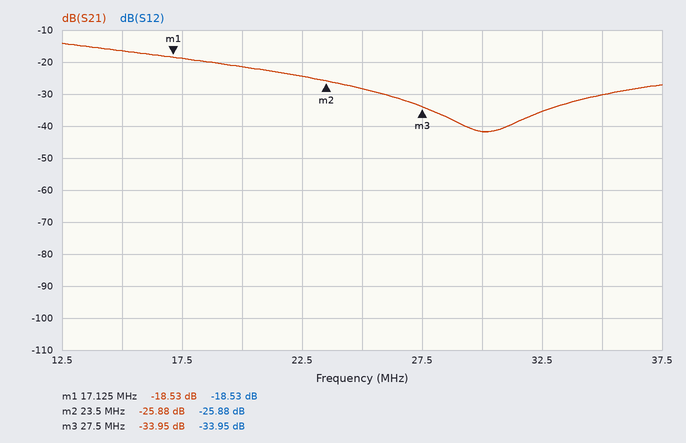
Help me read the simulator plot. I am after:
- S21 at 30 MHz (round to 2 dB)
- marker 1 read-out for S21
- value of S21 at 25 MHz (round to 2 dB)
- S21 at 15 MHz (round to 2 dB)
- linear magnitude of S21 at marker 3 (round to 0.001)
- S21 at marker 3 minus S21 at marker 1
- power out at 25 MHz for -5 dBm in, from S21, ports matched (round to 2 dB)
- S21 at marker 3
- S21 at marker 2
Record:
-42 dB
-18.53 dB
-28 dB
-16 dB
0.020
-15.42 dB
-34 dBm
-33.95 dB
-25.88 dB
